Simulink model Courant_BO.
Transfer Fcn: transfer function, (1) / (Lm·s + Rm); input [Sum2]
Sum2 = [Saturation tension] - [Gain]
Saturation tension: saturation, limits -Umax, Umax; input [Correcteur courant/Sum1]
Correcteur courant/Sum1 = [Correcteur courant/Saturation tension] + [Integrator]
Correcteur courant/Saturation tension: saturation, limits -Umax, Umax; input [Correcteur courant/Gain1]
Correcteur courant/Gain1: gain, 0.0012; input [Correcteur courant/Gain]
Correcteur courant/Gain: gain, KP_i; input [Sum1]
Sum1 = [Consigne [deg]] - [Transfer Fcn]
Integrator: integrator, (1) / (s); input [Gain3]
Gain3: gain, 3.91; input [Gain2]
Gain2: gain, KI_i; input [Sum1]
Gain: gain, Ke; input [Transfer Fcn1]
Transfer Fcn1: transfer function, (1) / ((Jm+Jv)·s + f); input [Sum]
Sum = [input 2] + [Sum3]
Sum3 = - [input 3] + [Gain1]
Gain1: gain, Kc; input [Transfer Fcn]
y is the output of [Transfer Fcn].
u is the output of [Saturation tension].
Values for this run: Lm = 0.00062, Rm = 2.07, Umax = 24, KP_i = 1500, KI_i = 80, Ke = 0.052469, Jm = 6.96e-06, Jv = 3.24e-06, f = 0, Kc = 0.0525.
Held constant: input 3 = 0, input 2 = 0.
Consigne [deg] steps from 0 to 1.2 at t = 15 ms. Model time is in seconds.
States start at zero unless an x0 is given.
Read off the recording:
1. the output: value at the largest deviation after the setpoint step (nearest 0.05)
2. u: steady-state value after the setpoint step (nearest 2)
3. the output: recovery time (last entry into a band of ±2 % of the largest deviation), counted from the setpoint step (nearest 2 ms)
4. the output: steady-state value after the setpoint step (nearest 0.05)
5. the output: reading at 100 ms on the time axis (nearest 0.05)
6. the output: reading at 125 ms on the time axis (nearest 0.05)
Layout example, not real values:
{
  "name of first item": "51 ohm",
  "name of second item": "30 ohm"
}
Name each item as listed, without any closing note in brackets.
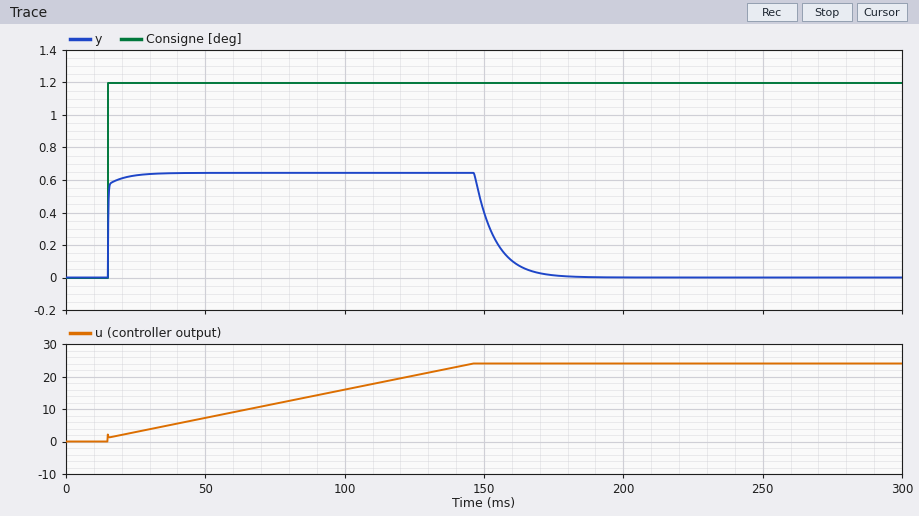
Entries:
{
  "the output: value at the largest deviation after the setpoint step": "0.65",
  "u: steady-state value after the setpoint step": "24",
  "the output: recovery time (last entry into a band of ±2 % of the largest deviation), counted from the setpoint step": "160 ms",
  "the output: steady-state value after the setpoint step": "0.00",
  "the output: reading at 100 ms on the time axis": "0.65",
  "the output: reading at 125 ms on the time axis": "0.65"
}
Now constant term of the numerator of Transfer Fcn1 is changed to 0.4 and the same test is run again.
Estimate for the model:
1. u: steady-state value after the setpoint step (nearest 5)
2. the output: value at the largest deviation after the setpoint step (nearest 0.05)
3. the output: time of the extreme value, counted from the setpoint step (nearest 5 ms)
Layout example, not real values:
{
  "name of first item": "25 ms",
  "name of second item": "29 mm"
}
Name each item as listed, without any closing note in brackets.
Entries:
{
  "u: steady-state value after the setpoint step": "25",
  "the output: value at the largest deviation after the setpoint step": "0.90",
  "the output: time of the extreme value, counted from the setpoint step": "235 ms"
}
